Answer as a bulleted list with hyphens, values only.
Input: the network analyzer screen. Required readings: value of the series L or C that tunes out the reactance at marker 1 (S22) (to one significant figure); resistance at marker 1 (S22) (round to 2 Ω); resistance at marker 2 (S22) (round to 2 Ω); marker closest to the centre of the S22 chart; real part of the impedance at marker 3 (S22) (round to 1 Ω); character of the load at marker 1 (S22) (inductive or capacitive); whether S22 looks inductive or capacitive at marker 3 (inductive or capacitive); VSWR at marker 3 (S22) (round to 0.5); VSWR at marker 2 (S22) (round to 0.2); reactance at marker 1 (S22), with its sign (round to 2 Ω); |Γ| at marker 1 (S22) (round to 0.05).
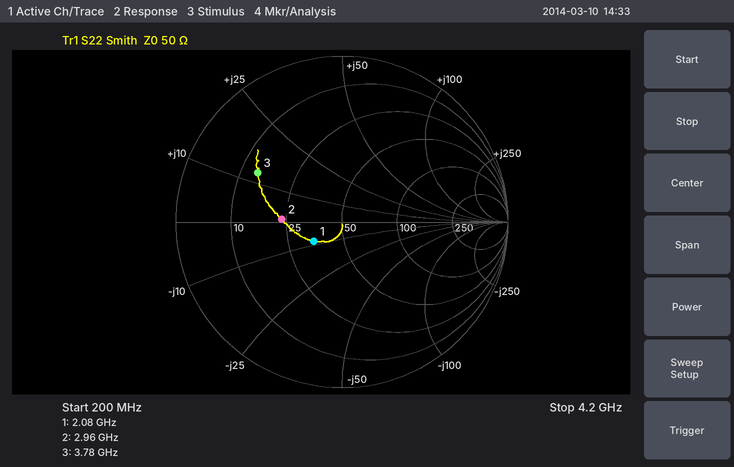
- 600 pH
- 34 Ω
- 24 Ω
- marker 1
- 14 Ω
- capacitive
- inductive
- 4.0
- 2.2
- -8 Ω
- 0.20
